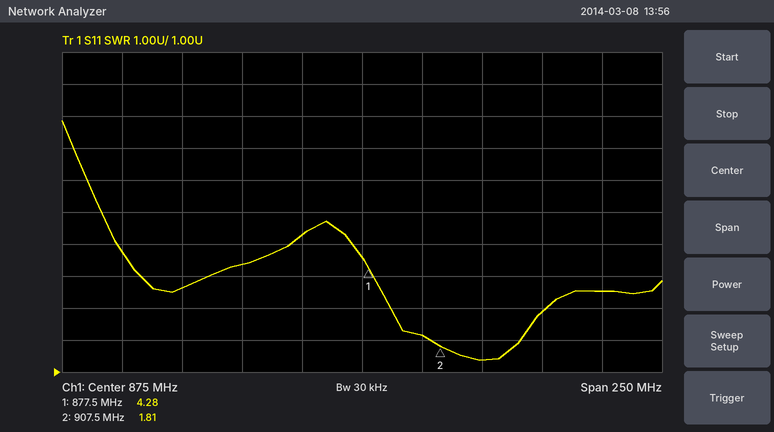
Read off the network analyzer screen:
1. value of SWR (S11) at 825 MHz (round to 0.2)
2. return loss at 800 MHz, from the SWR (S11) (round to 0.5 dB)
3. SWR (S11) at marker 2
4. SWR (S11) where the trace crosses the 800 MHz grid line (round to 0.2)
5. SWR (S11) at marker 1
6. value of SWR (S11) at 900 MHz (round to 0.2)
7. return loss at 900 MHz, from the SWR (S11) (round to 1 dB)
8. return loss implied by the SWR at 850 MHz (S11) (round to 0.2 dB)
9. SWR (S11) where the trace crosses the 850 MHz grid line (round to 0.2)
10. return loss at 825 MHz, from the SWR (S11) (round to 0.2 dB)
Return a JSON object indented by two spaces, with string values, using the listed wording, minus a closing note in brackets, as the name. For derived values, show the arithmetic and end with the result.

{
  "value of SWR (S11) at 825 MHz": "4.4",
  "return loss at 800 MHz, from the SWR (S11)": "−20 log10((3.6 − 1)/(3.6 + 1)) ≈ 5.0 dB",
  "SWR (S11) at marker 2": "1.81",
  "SWR (S11) where the trace crosses the 800 MHz grid line": "3.6",
  "SWR (S11) at marker 1": "4.28",
  "value of SWR (S11) at 900 MHz": "2.2",
  "return loss at 900 MHz, from the SWR (S11)": "−20 log10((2.2 − 1)/(2.2 + 1)) ≈ 9 dB",
  "return loss implied by the SWR at 850 MHz (S11)": "−20 log10((5.2 − 1)/(5.2 + 1)) ≈ 3.4 dB",
  "SWR (S11) where the trace crosses the 850 MHz grid line": "5.2",
  "return loss at 825 MHz, from the SWR (S11)": "−20 log10((4.4 − 1)/(4.4 + 1)) ≈ 4.0 dB"
}
